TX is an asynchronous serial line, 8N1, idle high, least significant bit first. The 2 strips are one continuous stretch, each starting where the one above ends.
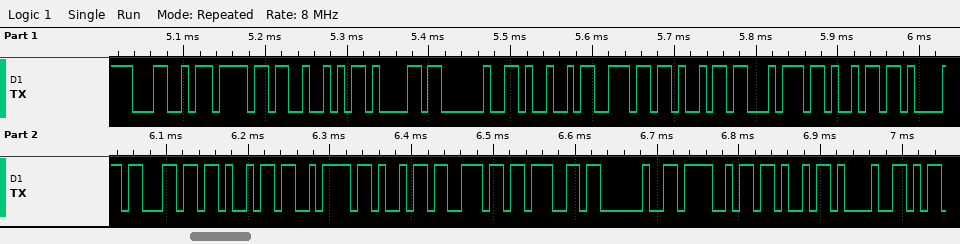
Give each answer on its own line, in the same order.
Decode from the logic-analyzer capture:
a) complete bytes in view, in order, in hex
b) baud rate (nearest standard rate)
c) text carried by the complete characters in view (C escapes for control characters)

4C 6F 52 61 20 49 6E 69 74 69 61 6C 69 7A 69 6E 67 20 4F 4B 21
115200 baud
"LoRa Initializing OK!"
